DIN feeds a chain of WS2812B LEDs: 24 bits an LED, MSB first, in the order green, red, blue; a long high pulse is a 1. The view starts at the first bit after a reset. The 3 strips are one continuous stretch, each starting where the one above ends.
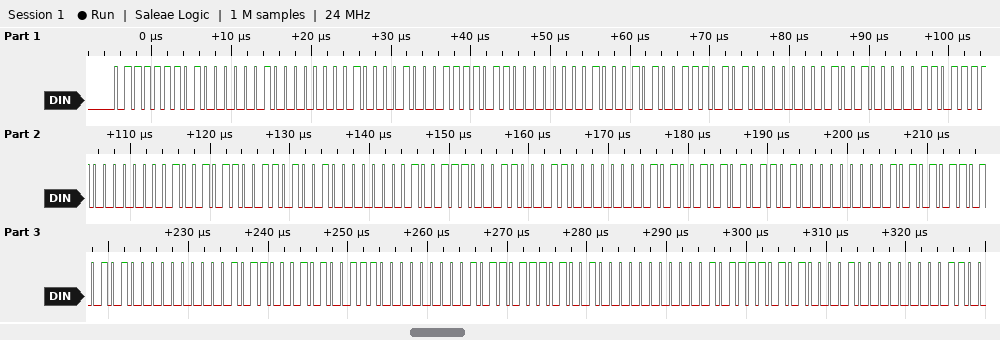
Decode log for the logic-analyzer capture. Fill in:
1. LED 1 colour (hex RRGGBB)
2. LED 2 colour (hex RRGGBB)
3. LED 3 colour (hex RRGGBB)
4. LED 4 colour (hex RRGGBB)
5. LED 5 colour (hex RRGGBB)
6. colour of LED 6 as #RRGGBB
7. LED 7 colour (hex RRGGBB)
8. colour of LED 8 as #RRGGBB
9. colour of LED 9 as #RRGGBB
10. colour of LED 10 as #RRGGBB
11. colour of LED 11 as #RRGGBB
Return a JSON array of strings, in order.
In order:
["#817E00", "#7B8400", "#758A00", "#6F9000", "#699600", "#639C00", "#5AA500", "#54AB00", "#4EB100", "#48B700", "#42BD00"]
